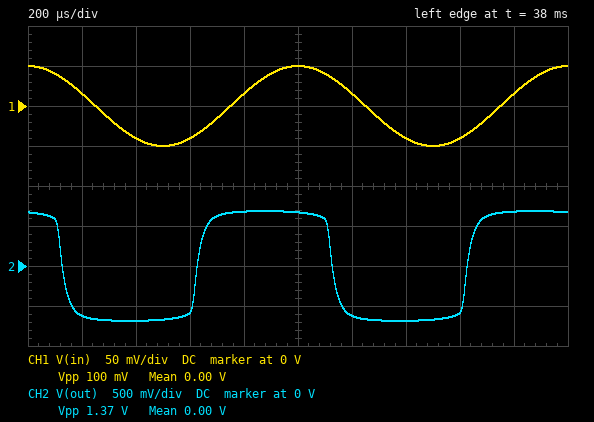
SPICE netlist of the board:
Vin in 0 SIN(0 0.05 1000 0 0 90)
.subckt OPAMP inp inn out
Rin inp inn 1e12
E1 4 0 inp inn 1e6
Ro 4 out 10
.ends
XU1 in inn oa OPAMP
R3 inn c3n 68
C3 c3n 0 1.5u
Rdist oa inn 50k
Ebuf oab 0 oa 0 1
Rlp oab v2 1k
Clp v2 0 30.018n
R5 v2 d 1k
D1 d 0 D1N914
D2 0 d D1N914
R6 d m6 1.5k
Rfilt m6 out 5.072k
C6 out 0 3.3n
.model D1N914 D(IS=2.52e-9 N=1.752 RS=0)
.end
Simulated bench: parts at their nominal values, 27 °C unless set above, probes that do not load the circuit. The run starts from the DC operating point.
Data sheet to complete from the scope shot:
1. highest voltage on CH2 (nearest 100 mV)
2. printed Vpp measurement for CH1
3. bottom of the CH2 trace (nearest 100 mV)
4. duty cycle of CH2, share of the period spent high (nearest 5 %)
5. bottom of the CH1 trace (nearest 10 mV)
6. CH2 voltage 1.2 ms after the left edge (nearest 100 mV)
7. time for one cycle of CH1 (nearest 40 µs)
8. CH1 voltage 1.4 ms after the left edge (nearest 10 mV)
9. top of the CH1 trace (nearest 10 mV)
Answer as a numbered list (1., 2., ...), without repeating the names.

1. 700 mV
2. 100 mV
3. -700 mV
4. 50 %
5. -50 mV
6. -600 mV
7. 1.00 ms
8. -40 mV
9. 50 mV
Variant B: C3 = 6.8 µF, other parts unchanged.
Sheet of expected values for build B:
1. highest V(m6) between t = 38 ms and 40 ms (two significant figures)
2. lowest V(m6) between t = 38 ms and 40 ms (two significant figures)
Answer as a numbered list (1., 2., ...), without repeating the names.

1. 710 mV
2. -710 mV
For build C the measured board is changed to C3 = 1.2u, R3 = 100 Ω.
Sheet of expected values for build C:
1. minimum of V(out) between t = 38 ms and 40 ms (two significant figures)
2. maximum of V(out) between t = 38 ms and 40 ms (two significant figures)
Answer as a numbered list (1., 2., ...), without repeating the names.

1. -670 mV
2. 670 mV
